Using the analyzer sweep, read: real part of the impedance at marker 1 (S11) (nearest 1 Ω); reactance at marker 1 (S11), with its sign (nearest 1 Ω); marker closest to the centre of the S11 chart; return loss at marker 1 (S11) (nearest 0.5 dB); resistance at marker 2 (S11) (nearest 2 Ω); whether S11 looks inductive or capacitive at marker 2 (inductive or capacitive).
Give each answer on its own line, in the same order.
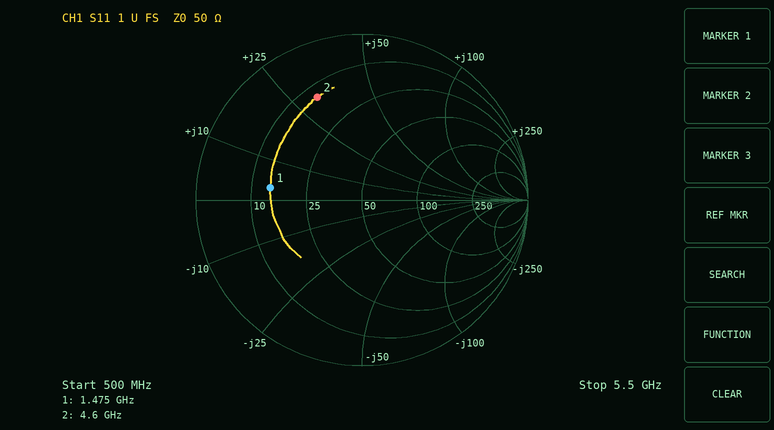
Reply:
14 Ω
+3 Ω
marker 1
5.0 dB
14 Ω
inductive
